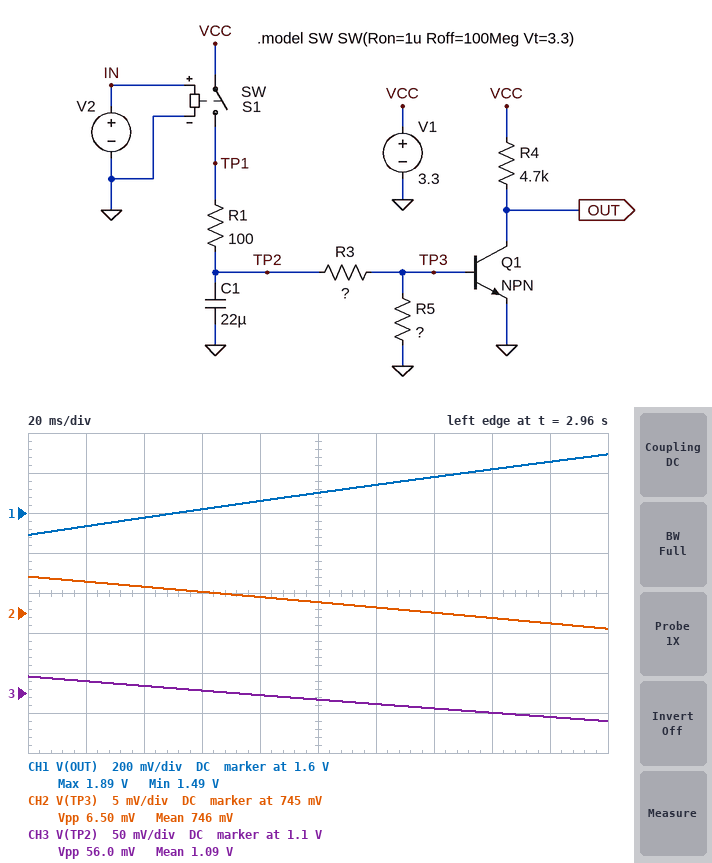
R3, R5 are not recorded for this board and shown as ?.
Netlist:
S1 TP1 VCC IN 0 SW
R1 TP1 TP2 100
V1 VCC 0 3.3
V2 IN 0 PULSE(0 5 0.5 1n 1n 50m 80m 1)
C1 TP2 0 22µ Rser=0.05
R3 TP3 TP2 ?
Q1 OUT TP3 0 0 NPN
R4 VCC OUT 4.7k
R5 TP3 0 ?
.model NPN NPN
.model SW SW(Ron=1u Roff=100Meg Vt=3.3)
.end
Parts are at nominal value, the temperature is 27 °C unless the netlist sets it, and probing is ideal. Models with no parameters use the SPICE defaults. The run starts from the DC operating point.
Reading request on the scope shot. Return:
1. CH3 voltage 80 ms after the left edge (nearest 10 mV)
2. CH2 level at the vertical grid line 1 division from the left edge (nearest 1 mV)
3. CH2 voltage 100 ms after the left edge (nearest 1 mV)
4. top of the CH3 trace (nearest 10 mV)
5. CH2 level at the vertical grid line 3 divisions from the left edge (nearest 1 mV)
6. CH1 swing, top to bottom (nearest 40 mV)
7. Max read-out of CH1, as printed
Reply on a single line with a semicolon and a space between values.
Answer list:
1.10 V; 749 mV; 746 mV; 1.12 V; 748 mV; 400 mV; 1.89 V
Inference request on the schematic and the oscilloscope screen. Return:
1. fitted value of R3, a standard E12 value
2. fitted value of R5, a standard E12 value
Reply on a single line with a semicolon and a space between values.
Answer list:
56 kΩ; 270 kΩ
